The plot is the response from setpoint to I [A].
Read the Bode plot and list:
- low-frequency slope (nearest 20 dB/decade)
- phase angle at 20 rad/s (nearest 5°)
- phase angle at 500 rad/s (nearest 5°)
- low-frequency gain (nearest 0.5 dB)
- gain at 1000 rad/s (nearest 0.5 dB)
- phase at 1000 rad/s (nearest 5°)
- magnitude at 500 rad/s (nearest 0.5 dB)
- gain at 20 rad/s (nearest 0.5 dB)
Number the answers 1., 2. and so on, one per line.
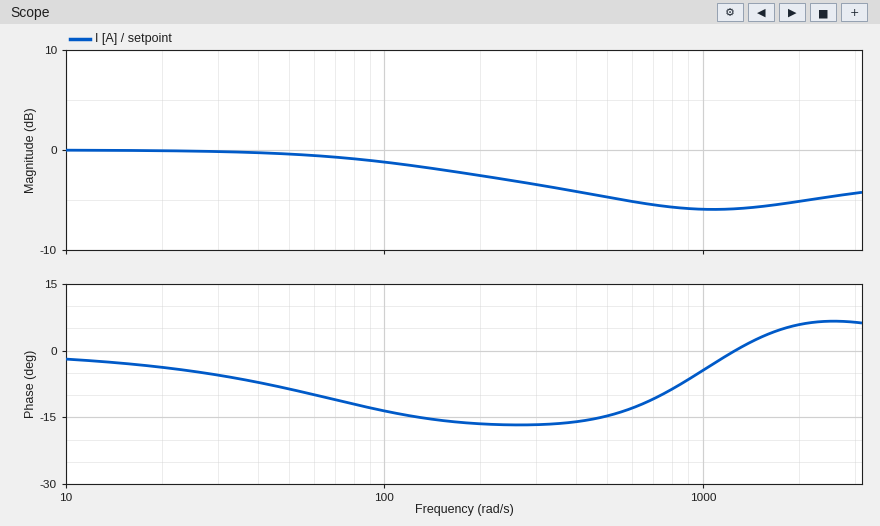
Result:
1. 0 dB/decade
2. -5°
3. -15°
4. 0.0 dB
5. -6.0 dB
6. -5°
7. -4.5 dB
8. 0.0 dB
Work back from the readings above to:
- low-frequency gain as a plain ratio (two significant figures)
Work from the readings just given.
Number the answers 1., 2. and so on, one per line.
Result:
1. 1.0
